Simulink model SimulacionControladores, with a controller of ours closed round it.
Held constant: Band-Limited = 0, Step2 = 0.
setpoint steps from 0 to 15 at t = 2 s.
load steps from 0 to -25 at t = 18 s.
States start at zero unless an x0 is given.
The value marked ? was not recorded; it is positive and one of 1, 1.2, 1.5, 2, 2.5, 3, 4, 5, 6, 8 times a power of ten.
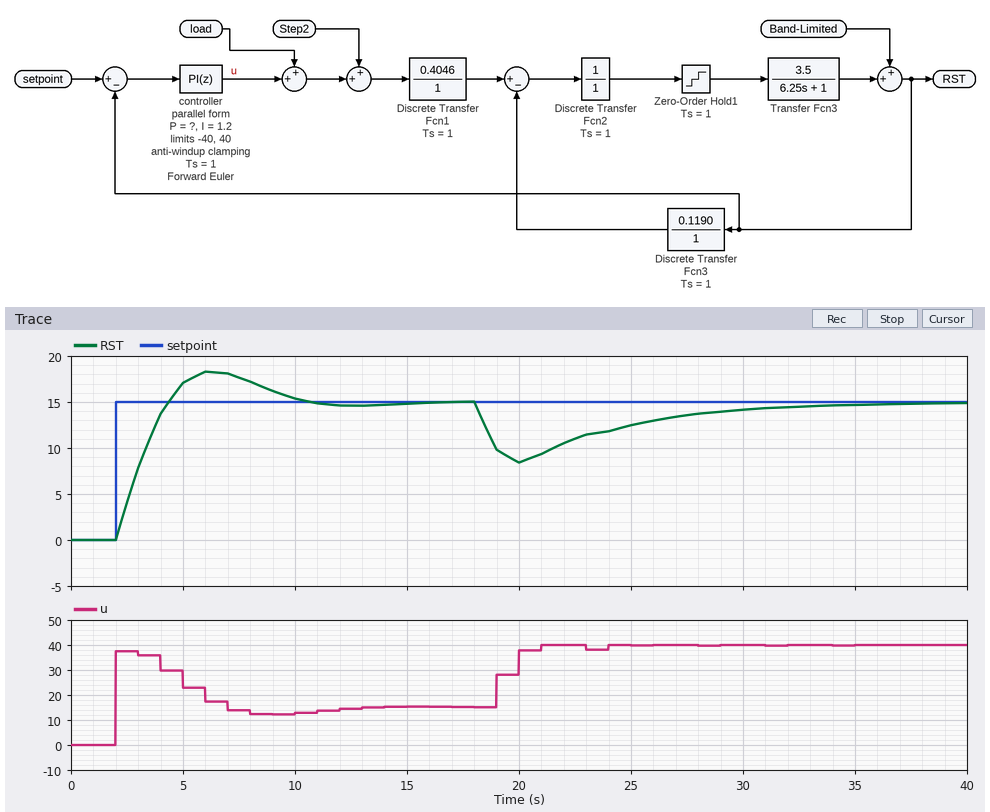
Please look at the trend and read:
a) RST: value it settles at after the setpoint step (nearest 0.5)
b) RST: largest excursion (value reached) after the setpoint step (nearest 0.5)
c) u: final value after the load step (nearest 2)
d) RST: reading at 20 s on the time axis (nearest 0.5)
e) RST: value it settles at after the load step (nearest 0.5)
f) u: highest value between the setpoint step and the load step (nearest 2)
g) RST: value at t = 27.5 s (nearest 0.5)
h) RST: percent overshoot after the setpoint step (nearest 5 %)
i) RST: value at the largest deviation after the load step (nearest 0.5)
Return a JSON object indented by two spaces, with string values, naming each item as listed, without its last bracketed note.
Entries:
{
  "RST: value it settles at after the setpoint step": "15.0",
  "RST: largest excursion (value reached) after the setpoint step": "18.5",
  "u: final value after the load step": "40",
  "RST: reading at 20 s on the time axis": "8.5",
  "RST: value it settles at after the load step": "15.0",
  "u: highest value between the setpoint step and the load step": "38",
  "RST: value at t = 27.5 s": "13.5",
  "RST: percent overshoot after the setpoint step": "20 %",
  "RST: value at the largest deviation after the load step": "8.5"
}
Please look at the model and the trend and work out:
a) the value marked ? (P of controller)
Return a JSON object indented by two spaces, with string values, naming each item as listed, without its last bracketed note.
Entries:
{
  "the value marked ?": "2.5"
}
